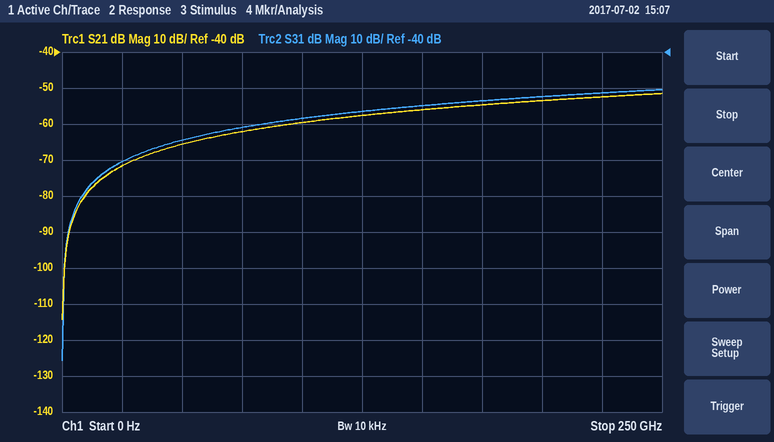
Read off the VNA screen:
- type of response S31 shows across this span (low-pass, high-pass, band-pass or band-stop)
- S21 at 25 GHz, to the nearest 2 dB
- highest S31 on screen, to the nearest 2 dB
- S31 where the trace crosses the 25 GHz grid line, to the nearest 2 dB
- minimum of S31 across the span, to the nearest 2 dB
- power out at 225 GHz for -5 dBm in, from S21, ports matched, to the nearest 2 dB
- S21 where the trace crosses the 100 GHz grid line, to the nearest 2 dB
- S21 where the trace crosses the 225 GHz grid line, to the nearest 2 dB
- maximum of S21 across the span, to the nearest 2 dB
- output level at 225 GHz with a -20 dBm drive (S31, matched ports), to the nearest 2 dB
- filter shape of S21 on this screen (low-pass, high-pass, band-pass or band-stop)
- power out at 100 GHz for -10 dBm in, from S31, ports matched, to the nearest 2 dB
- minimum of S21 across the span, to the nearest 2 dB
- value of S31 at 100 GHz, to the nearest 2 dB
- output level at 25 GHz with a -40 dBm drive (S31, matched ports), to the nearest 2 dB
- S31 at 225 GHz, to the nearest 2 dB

high-pass
-72 dB
-50 dB
-70 dB
-126 dB
-58 dBm
-60 dB
-52 dB
-52 dB
-72 dBm
high-pass
-68 dBm
-114 dB
-58 dB
-110 dBm
-52 dB
